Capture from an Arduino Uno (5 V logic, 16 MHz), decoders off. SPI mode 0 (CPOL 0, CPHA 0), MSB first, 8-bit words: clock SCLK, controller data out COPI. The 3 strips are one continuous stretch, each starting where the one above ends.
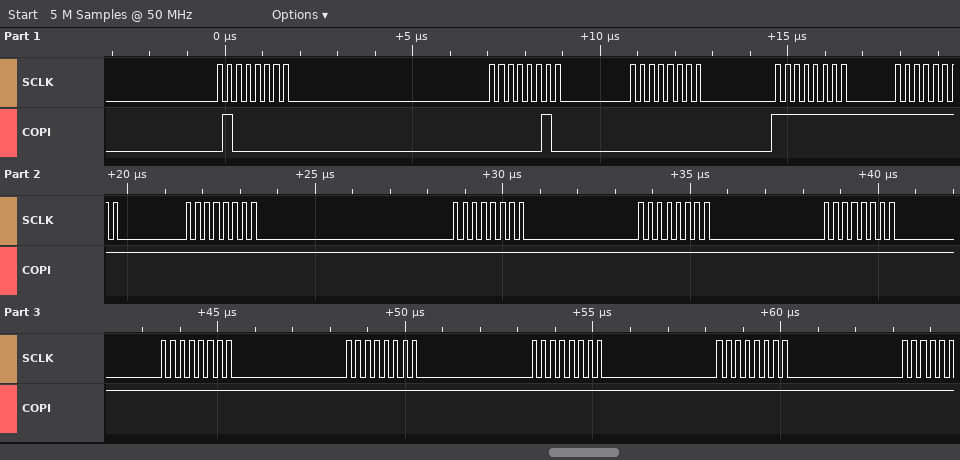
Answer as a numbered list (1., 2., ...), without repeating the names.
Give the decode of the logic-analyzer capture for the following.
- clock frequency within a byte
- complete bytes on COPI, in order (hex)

1. 4 MHz
2. 40 02 00 FF FF FF FF FF FF FF FF FF FF
